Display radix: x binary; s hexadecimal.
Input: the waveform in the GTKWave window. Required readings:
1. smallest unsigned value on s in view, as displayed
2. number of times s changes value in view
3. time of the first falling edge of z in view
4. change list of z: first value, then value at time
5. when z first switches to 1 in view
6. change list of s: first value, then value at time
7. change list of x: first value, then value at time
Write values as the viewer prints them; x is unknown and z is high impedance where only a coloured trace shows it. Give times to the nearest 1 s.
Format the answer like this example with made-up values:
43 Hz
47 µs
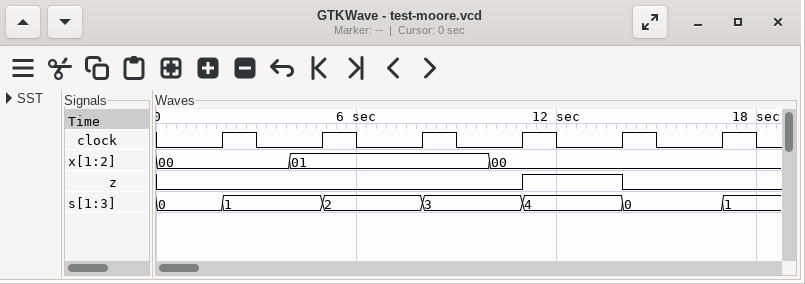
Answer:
0
6
14 s
0, 1 at 11 s, 0 at 14 s
11 s
0, 1 at 2 s, 2 at 5 s, 3 at 8 s, 4 at 11 s, 0 at 14 s, 1 at 17 s
00, 01 at 4 s, 00 at 10 s
